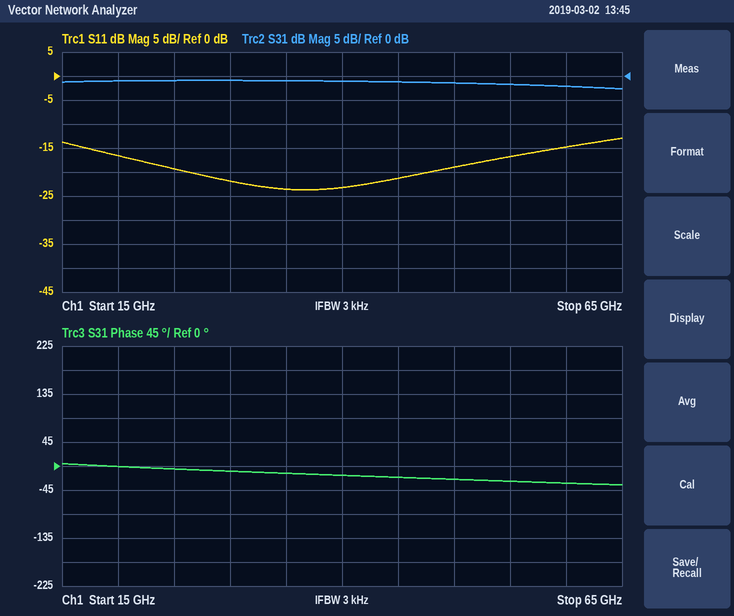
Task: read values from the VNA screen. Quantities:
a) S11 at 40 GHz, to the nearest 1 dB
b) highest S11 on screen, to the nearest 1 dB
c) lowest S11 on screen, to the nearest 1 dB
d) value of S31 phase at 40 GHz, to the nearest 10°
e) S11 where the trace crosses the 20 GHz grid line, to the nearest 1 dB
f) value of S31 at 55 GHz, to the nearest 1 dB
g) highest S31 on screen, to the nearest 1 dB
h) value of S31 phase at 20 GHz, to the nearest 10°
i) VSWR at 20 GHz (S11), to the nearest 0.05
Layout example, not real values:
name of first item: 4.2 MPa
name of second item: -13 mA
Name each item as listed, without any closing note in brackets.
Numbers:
S11 at 40 GHz, to the nearest 1 dB: -23 dB
highest S11 on screen, to the nearest 1 dB: -13 dB
lowest S11 on screen, to the nearest 1 dB: -24 dB
value of S31 phase at 40 GHz, to the nearest 10°: -20°
S11 where the trace crosses the 20 GHz grid line, to the nearest 1 dB: -17 dB
value of S31 at 55 GHz, to the nearest 1 dB: -2 dB
highest S31 on screen, to the nearest 1 dB: -1 dB
value of S31 phase at 20 GHz, to the nearest 10°: 0°
VSWR at 20 GHz (S11), to the nearest 0.05: 1.35
